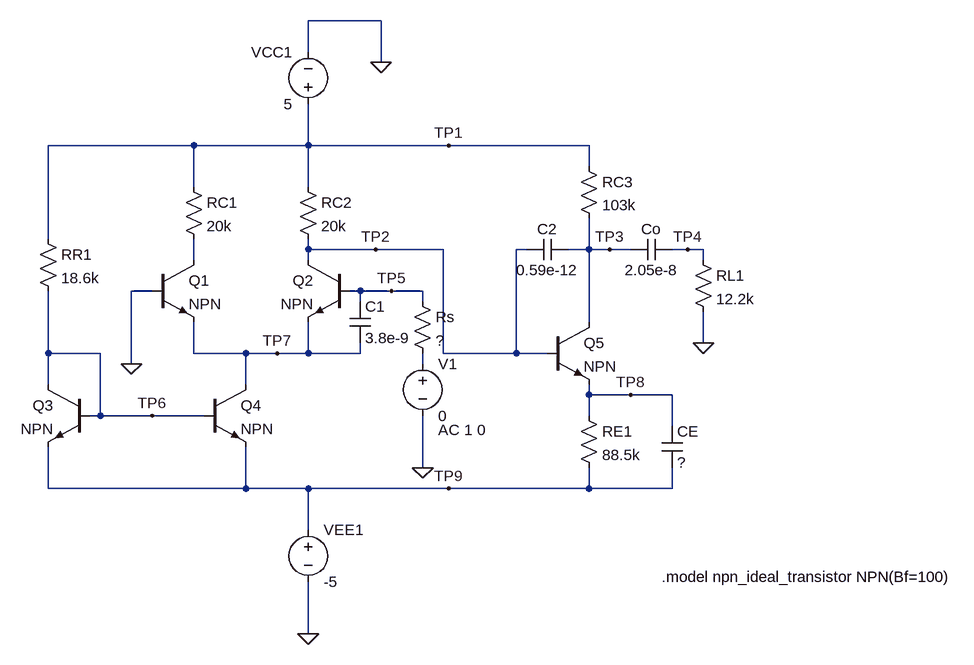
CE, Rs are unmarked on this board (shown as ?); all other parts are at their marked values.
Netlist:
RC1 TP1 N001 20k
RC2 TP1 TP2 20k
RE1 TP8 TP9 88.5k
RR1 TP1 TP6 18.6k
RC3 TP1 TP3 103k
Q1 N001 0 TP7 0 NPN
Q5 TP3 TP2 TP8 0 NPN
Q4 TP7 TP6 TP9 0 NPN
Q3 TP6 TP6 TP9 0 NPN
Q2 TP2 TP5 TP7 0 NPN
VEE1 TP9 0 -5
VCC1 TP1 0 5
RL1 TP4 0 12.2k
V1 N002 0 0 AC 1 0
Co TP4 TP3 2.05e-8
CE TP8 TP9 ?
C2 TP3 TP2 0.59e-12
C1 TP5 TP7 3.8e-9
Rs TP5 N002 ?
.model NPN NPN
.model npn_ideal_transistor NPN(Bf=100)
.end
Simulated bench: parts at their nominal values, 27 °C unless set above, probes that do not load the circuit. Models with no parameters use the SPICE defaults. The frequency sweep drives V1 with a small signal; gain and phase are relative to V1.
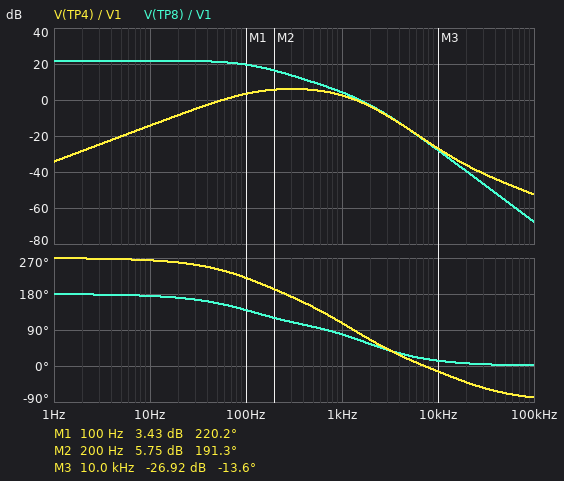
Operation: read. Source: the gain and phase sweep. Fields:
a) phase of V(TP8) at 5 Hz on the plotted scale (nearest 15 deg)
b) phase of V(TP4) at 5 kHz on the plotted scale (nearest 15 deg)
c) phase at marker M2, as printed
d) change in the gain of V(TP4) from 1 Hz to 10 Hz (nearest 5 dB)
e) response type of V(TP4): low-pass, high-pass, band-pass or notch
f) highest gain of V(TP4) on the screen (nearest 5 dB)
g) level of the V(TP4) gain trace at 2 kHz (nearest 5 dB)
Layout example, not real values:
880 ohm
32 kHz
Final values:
180 deg
15 deg
191.3 deg
20 dB
band-pass
5 dB
-5 dB
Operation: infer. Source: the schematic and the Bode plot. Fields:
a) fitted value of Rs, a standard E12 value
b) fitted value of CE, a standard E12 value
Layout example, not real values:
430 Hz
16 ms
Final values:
68 kΩ
68 nF
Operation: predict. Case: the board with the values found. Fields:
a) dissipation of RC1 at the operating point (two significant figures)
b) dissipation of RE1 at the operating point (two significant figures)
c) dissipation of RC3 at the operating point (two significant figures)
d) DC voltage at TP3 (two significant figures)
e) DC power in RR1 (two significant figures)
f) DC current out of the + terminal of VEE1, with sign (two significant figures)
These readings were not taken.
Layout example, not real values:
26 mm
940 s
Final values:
1.6 mW
530 µW
95 µW
1.9 V
4.6 mW
-1.1 mA
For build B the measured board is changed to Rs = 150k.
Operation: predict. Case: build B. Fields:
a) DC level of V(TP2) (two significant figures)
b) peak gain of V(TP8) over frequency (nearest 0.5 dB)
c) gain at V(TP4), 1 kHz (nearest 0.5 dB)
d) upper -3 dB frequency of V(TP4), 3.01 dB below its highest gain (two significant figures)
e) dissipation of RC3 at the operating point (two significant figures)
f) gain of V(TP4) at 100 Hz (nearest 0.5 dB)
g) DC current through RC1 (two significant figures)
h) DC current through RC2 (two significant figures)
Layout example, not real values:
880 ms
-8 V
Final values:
3.0 V
16.0 dB
-5.0 dB
760 Hz
71 µW
-2.5 dB
290 µA
100 µA
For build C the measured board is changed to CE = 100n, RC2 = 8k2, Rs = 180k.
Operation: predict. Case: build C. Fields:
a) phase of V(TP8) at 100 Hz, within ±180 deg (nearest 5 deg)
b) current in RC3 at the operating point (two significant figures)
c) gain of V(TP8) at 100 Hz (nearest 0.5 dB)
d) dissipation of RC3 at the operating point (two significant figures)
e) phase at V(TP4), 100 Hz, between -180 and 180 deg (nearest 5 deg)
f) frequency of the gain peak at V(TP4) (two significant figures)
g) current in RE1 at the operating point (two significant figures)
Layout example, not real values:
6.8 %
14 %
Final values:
145 deg
16 µA
7.5 dB
27 µW
-135 deg
310 Hz
94 µA
